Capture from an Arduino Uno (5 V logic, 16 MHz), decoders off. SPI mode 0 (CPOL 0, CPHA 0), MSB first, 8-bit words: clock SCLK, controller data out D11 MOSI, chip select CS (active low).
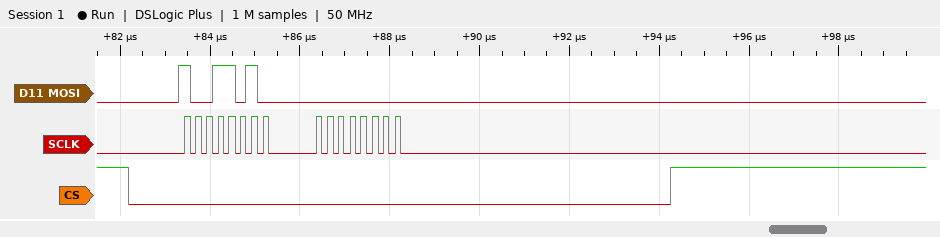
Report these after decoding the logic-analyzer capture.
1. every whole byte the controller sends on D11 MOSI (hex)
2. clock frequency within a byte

9A 00
4 MHz
